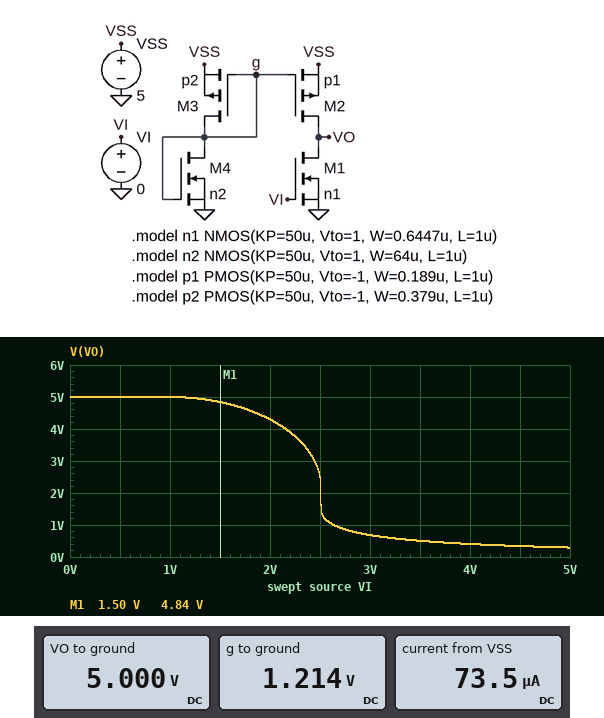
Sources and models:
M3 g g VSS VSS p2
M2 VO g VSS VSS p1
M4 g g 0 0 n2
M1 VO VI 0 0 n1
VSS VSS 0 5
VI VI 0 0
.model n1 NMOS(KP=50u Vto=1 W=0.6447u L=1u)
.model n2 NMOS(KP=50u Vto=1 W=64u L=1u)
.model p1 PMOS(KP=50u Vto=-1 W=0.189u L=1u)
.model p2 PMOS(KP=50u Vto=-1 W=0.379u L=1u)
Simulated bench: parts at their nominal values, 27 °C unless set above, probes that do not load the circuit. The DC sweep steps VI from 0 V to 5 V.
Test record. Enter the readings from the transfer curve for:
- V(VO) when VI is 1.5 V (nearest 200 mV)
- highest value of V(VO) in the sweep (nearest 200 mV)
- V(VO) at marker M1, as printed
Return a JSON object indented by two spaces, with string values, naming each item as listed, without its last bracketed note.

{
  "V(VO) when VI is 1.5 V": "4.8 V",
  "highest value of V(VO) in the sweep": "5.0 V",
  "V(VO) at marker M1, as printed": "4.84 V"
}
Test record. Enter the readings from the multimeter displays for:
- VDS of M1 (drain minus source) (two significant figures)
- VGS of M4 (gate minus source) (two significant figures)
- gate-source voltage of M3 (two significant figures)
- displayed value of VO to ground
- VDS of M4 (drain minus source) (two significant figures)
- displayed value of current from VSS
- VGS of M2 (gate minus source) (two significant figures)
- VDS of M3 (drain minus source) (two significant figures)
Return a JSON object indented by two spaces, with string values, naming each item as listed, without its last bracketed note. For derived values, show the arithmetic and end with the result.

{
  "VDS of M1 (drain minus source)": "5 V = 5.0 V",
  "VGS of M4 (gate minus source)": "1.214 V = 1.2 V",
  "gate-source voltage of M3": "1.214 V - 5 V = -3.8 V",
  "displayed value of VO to ground": "5.000 V",
  "VDS of M4 (drain minus source)": "1.214 V = 1.2 V",
  "displayed value of current from VSS": "73.5 µA",
  "VGS of M2 (gate minus source)": "1.214 V - 5 V = -3.8 V",
  "VDS of M3 (drain minus source)": "1.214 V - 5 V = -3.8 V"
}
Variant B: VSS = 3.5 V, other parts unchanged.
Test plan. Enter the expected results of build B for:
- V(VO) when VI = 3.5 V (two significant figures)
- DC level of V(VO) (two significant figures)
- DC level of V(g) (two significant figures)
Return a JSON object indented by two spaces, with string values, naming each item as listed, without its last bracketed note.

{
  "V(VO) when VI = 3.5 V": "120 mV",
  "DC level of V(VO)": "3.5 V",
  "DC level of V(g)": "1.1 V"
}
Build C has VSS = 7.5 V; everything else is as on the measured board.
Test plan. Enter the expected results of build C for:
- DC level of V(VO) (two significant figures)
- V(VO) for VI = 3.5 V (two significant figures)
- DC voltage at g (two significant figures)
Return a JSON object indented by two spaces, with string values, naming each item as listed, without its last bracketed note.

{
  "DC level of V(VO)": "7.5 V",
  "V(VO) for VI = 3.5 V": "4.6 V",
  "DC voltage at g": "1.4 V"
}
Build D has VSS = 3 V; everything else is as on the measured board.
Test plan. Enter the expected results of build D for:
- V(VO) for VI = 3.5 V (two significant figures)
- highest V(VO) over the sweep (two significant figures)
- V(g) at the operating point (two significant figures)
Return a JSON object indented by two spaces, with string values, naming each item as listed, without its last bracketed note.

{
  "V(VO) for VI = 3.5 V": "51 mV",
  "highest V(VO) over the sweep": "3.0 V",
  "V(g) at the operating point": "1.1 V"
}
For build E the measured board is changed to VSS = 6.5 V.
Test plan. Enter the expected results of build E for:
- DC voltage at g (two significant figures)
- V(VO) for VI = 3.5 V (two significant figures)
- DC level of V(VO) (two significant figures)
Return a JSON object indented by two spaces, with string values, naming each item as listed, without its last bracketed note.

{
  "DC voltage at g": "1.3 V",
  "V(VO) for VI = 3.5 V": "1.4 V",
  "DC level of V(VO)": "6.5 V"
}
